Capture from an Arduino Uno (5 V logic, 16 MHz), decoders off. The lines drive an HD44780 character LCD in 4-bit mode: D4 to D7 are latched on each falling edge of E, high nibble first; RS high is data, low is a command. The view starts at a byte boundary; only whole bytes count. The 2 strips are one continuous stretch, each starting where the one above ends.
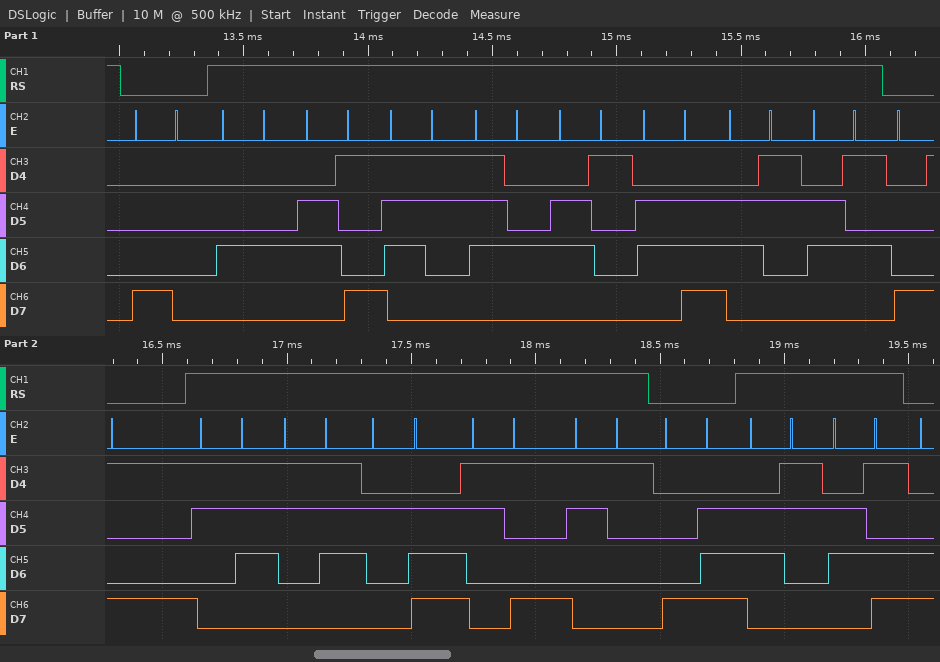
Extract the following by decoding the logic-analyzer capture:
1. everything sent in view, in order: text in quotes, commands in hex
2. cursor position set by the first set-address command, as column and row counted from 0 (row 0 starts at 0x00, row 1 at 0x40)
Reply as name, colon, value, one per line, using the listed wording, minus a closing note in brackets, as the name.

everything sent in view, in order: text in quotes, commands in hex: 0x80 "Distance" 0x89 "77.91" 0x8E "cm"
cursor position set by the first set-address command, as column and row counted from 0: column 0, row 0
